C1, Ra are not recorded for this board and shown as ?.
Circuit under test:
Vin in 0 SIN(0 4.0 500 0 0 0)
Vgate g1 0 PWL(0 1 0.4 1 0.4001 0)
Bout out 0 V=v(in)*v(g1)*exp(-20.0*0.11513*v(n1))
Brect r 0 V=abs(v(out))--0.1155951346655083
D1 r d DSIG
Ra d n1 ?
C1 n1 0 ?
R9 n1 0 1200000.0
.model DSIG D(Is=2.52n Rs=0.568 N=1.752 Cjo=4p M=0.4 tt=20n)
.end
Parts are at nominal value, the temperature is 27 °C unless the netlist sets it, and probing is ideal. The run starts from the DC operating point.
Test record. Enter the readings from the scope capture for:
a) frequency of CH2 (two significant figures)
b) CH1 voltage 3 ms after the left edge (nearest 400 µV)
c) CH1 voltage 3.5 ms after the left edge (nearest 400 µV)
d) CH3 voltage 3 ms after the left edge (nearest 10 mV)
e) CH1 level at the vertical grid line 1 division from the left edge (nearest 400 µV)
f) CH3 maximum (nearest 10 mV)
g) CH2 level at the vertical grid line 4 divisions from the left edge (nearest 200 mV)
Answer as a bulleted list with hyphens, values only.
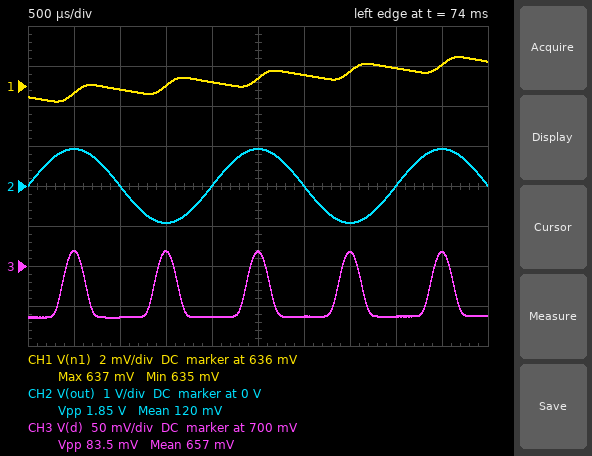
- 500 Hz
- 636.4 mV
- 636.8 mV
- 640 mV
- 635.6 mV
- 720 mV
- 0 V
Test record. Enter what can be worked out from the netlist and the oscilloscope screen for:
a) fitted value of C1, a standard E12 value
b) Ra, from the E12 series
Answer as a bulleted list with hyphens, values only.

- 680 nF
- 27 kΩ
